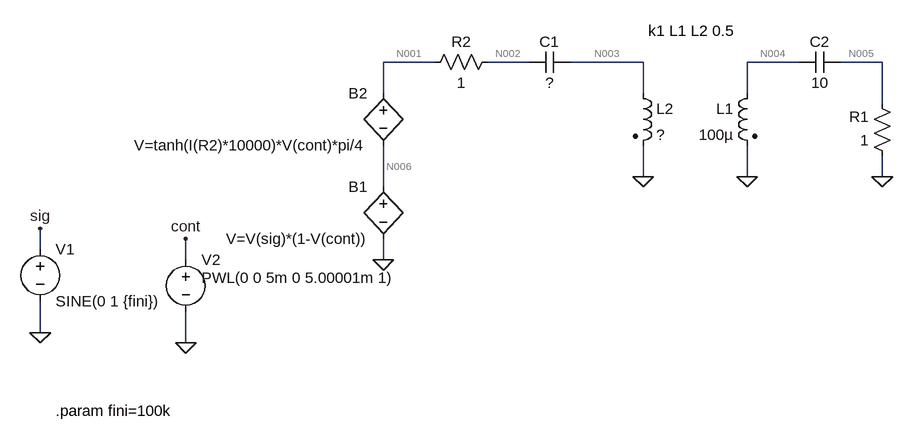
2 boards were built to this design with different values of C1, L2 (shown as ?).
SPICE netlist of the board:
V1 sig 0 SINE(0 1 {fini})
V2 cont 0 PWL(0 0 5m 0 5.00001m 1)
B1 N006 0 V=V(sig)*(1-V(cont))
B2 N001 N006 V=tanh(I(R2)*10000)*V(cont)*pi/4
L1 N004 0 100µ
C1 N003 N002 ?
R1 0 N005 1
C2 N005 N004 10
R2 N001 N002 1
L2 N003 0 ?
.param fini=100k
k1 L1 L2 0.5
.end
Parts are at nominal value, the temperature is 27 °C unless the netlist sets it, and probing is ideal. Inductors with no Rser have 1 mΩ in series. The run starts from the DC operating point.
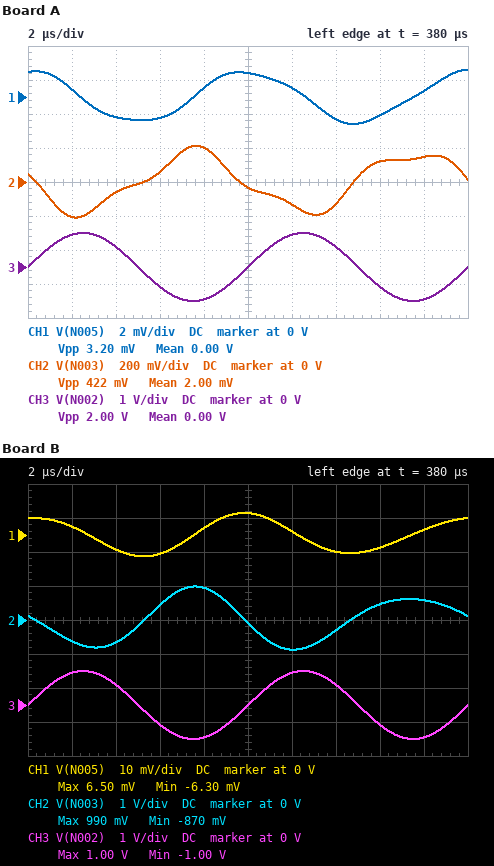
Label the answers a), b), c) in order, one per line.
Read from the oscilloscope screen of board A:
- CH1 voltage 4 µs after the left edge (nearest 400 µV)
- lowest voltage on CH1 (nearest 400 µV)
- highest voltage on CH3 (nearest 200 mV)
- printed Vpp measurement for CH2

a) -1.2 mV
b) -1.6 mV
c) 1.0 V
d) 422 mV
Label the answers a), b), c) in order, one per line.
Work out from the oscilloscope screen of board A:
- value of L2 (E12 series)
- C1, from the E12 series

a) 150 µH
b) 3.3 nF
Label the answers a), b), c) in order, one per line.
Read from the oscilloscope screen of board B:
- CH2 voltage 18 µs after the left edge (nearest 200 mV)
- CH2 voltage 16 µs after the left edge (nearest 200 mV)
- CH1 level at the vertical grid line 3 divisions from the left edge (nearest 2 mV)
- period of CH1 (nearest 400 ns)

a) 600 mV
b) 400 mV
c) -6 mV
d) 10.0 µs
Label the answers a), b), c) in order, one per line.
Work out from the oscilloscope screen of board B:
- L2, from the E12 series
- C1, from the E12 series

a) 220 µH
b) 6.8 nF
